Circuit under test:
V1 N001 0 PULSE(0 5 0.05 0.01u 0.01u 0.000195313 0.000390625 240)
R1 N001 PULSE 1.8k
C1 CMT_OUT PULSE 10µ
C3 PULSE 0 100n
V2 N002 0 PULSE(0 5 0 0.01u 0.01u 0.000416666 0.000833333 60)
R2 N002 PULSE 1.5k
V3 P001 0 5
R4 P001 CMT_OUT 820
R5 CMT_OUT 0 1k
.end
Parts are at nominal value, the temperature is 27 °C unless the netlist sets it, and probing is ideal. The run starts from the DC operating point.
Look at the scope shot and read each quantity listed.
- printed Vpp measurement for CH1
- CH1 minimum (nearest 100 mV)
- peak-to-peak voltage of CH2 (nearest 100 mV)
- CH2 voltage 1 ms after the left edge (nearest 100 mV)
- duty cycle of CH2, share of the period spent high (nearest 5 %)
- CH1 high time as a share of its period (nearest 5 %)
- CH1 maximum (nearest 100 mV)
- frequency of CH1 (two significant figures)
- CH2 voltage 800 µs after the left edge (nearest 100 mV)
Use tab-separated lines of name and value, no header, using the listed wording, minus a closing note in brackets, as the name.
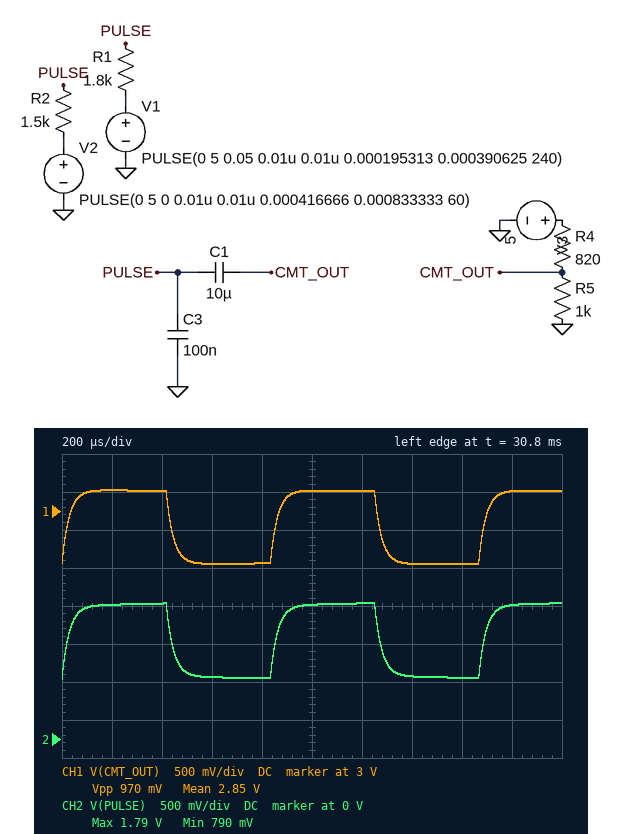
printed Vpp measurement for CH1	970 mV
CH1 minimum	2.3 V
peak-to-peak voltage of CH2	1.0 V
CH2 voltage 1 ms after the left edge	1.8 V
duty cycle of CH2, share of the period spent high	50 %
CH1 high time as a share of its period	50 %
CH1 maximum	3.3 V
frequency of CH1	1.2 kHz
CH2 voltage 800 µs after the left edge	800 mV
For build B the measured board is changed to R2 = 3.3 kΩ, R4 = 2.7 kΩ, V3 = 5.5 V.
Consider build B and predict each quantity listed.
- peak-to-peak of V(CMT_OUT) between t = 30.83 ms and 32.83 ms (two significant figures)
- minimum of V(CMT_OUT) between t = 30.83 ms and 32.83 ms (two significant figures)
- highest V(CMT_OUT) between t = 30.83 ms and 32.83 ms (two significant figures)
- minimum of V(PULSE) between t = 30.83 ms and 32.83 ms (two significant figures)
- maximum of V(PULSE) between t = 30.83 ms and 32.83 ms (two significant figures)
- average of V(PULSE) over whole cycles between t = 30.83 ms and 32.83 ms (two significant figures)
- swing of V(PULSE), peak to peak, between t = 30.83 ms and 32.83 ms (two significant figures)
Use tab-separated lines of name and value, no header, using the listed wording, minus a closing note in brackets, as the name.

peak-to-peak of V(CMT_OUT) between t = 30.83 ms and 32.83 ms	680 mV
minimum of V(CMT_OUT) between t = 30.83 ms and 32.83 ms	1.2 V
highest V(CMT_OUT) between t = 30.83 ms and 32.83 ms	1.9 V
minimum of V(PULSE) between t = 30.83 ms and 32.83 ms	430 mV
maximum of V(PULSE) between t = 30.83 ms and 32.83 ms	1.1 V
average of V(PULSE) over whole cycles between t = 30.83 ms and 32.83 ms	780 mV
swing of V(PULSE), peak to peak, between t = 30.83 ms and 32.83 ms	690 mV
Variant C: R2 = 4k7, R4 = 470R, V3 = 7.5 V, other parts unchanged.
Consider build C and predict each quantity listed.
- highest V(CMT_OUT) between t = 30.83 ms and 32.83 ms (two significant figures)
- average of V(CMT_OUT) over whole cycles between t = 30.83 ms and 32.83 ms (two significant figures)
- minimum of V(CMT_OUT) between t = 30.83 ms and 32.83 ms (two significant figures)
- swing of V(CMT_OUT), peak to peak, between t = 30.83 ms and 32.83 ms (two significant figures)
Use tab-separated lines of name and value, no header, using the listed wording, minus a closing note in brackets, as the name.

highest V(CMT_OUT) between t = 30.83 ms and 32.83 ms	5.3 V
average of V(CMT_OUT) over whole cycles between t = 30.83 ms and 32.83 ms	5.1 V
minimum of V(CMT_OUT) between t = 30.83 ms and 32.83 ms	5.0 V
swing of V(CMT_OUT), peak to peak, between t = 30.83 ms and 32.83 ms	270 mV
